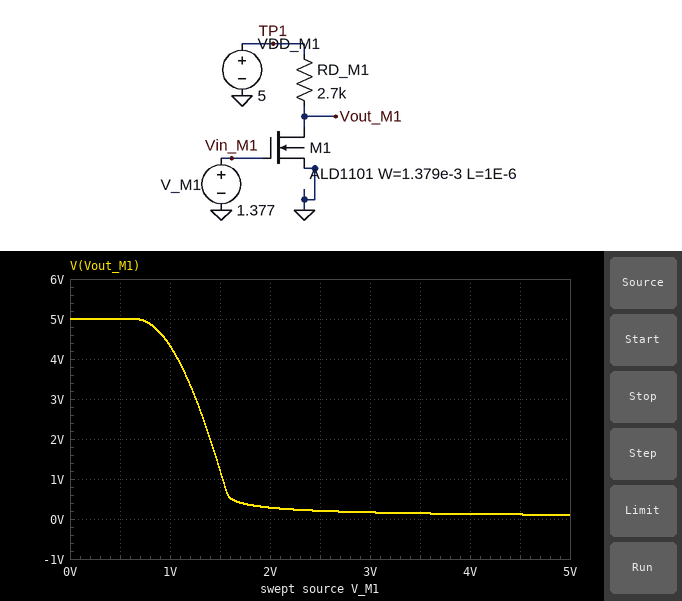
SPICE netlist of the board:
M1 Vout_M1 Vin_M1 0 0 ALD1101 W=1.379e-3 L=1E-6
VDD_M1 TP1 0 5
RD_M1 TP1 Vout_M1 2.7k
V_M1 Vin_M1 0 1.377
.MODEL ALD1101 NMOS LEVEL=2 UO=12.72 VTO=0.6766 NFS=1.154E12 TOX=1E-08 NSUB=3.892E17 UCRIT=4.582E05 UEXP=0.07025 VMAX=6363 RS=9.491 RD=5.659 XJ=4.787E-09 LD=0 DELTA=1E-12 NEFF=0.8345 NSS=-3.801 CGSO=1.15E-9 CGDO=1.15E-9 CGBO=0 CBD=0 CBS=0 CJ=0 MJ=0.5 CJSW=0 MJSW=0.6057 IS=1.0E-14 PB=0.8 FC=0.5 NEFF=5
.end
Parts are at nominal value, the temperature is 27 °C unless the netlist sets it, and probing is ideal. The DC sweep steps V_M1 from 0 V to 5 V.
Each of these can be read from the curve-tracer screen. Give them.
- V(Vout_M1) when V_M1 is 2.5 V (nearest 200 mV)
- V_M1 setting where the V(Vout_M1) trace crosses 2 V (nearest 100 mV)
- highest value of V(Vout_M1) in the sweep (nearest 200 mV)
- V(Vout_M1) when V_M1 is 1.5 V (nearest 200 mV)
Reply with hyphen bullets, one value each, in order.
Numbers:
- 200 mV
- 1.4 V
- 5.0 V
- 1.2 V
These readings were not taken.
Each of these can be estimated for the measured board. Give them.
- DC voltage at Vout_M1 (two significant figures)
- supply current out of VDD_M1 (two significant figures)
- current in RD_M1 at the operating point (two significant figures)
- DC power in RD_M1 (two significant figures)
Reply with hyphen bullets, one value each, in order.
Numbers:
- 2.2 V
- 1.0 mA
- 1.0 mA
- 2.9 mW
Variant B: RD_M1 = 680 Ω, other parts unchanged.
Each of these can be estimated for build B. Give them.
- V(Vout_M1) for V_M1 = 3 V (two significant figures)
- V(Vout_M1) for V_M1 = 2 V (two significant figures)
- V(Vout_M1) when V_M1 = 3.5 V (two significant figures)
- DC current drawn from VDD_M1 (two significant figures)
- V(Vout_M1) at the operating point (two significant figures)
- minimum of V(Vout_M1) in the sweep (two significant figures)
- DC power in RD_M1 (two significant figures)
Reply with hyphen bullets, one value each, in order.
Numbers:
- 690 mV
- 2.6 V
- 570 mV
- 1.1 mA
- 4.3 V
- 400 mV
- 770 µW
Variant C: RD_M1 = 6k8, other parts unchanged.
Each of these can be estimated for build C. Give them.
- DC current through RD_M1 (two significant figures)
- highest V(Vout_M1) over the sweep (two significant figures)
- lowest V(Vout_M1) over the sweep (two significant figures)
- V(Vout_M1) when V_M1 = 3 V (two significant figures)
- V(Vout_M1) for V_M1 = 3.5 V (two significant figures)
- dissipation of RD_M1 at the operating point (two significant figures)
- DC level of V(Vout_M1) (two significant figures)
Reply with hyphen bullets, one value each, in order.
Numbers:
- 700 µA
- 5.0 V
- 41 mV
- 65 mV
- 56 mV
- 3.4 mW
- 220 mV
